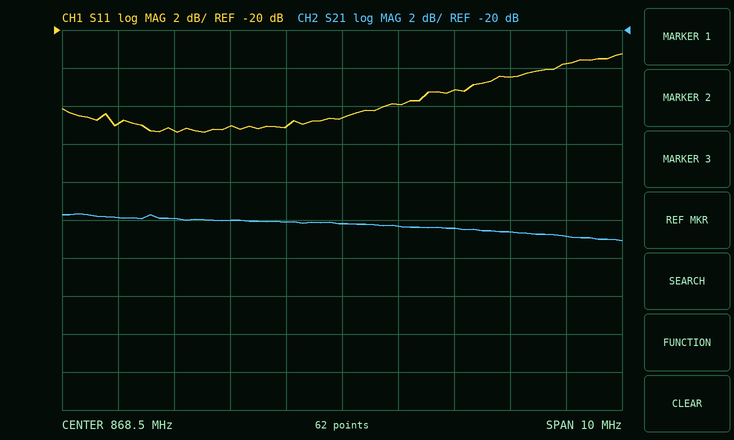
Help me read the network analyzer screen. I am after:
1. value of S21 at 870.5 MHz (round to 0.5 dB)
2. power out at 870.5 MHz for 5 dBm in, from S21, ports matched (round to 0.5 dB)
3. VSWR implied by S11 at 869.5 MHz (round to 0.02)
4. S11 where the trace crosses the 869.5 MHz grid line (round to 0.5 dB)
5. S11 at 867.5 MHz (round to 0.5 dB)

-30.5 dB
-25.5 dBm
1.14
-24.0 dB
-25.0 dB
